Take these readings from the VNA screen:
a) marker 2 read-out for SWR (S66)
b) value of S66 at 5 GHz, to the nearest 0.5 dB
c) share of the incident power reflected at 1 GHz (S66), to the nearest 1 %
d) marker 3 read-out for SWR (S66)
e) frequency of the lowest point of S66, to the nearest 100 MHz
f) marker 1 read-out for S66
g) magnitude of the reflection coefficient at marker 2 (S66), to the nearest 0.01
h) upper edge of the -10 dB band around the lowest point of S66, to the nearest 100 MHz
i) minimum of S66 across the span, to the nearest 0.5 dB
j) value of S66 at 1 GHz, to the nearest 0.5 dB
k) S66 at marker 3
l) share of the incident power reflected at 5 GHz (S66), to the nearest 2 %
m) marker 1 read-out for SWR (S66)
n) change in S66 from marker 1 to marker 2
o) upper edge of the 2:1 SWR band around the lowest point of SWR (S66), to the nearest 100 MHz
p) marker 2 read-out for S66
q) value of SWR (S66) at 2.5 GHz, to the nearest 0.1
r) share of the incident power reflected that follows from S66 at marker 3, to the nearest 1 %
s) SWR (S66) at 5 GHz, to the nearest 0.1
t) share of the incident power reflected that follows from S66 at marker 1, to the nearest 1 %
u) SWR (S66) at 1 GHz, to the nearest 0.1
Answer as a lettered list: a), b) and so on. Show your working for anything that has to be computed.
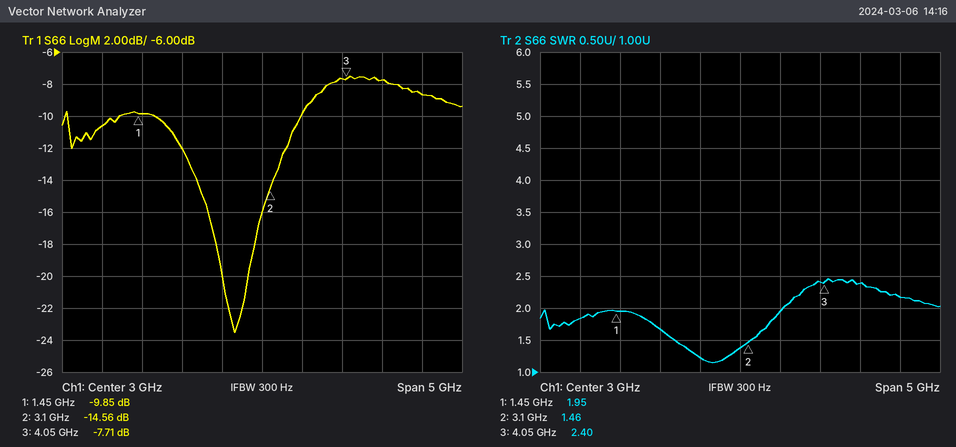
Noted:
a) 1.46
b) -8.5 dB
c) 10^(-10.5/10) ≈ 9 %
d) 2.40
e) 2.7 GHz
f) -9.85 dB
g) 10^(-14.56/20) ≈ 0.19
h) 3.5 GHz
i) -23.5 dB
j) -10.5 dB
k) -7.71 dB
l) 10^(-8.5/10) ≈ 14 %
m) 1.95
n) -14.56 − (-9.85) = -4.71 dB
o) 3.5 GHz
p) -14.56 dB
q) 1.2
r) 10^(-7.71/10) ≈ 17 %
s) 2.2
t) 10^(-9.85/10) ≈ 10 %
u) 1.8
